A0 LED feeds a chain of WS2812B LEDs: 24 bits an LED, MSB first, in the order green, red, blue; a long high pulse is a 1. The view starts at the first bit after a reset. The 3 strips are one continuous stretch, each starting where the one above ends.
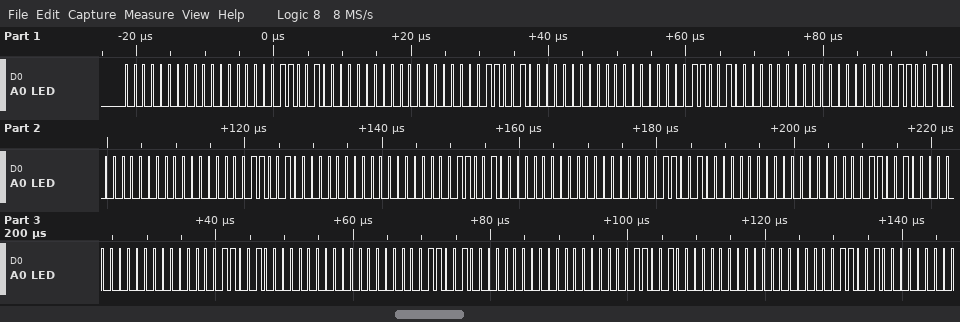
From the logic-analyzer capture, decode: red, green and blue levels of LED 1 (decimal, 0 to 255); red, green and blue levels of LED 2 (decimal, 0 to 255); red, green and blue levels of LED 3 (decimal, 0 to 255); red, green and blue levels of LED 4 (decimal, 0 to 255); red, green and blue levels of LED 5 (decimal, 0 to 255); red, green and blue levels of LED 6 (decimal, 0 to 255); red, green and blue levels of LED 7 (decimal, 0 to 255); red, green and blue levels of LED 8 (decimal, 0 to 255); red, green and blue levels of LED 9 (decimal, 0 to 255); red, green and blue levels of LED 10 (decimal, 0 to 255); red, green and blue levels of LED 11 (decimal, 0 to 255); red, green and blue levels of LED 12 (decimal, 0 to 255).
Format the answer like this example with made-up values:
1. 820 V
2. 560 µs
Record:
1. 0, 0, 50
2. 0, 0, 50
3. 0, 0, 50
4. 0, 0, 50
5. 0, 0, 50
6. 0, 0, 50
7. 0, 0, 50
8. 0, 0, 50
9. 0, 0, 50
10. 0, 0, 50
11. 0, 0, 50
12. 0, 0, 50
